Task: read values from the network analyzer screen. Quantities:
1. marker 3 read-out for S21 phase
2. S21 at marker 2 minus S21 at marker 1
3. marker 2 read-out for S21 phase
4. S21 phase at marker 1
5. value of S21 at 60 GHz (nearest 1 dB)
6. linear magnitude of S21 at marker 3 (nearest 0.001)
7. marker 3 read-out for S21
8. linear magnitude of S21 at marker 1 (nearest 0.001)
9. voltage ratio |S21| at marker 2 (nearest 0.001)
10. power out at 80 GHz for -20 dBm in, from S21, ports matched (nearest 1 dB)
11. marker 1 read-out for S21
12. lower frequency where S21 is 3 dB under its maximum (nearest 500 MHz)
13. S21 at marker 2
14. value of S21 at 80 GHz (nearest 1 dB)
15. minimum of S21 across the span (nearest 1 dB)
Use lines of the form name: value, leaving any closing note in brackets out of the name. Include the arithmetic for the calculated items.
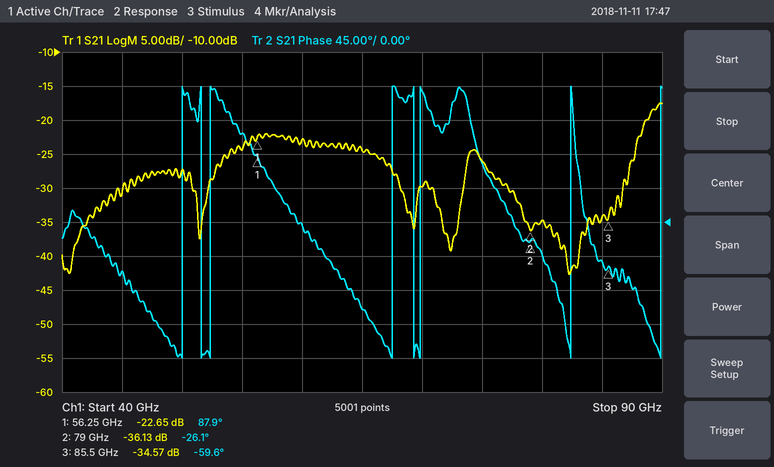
marker 3 read-out for S21 phase: -59.6°
S21 at marker 2 minus S21 at marker 1: -36.13 − (-22.65) = -13.48 dB
marker 2 read-out for S21 phase: -26.1°
S21 phase at marker 1: 87.9°
value of S21 at 60 GHz: -23 dB
linear magnitude of S21 at marker 3: 10^(-34.57/20) ≈ 0.019
marker 3 read-out for S21: -34.57 dB
linear magnitude of S21 at marker 1: 10^(-22.65/20) ≈ 0.074
voltage ratio |S21| at marker 2: 10^(-36.13/20) ≈ 0.016
power out at 80 GHz for -20 dBm in, from S21, ports matched: -20 dBm + (-35 dB) = -55 dBm
marker 1 read-out for S21: -22.65 dB
lower frequency where S21 is 3 dB under its maximum: 88.5 GHz
S21 at marker 2: -36.13 dB
value of S21 at 80 GHz: -35 dB
minimum of S21 across the span: -43 dB
